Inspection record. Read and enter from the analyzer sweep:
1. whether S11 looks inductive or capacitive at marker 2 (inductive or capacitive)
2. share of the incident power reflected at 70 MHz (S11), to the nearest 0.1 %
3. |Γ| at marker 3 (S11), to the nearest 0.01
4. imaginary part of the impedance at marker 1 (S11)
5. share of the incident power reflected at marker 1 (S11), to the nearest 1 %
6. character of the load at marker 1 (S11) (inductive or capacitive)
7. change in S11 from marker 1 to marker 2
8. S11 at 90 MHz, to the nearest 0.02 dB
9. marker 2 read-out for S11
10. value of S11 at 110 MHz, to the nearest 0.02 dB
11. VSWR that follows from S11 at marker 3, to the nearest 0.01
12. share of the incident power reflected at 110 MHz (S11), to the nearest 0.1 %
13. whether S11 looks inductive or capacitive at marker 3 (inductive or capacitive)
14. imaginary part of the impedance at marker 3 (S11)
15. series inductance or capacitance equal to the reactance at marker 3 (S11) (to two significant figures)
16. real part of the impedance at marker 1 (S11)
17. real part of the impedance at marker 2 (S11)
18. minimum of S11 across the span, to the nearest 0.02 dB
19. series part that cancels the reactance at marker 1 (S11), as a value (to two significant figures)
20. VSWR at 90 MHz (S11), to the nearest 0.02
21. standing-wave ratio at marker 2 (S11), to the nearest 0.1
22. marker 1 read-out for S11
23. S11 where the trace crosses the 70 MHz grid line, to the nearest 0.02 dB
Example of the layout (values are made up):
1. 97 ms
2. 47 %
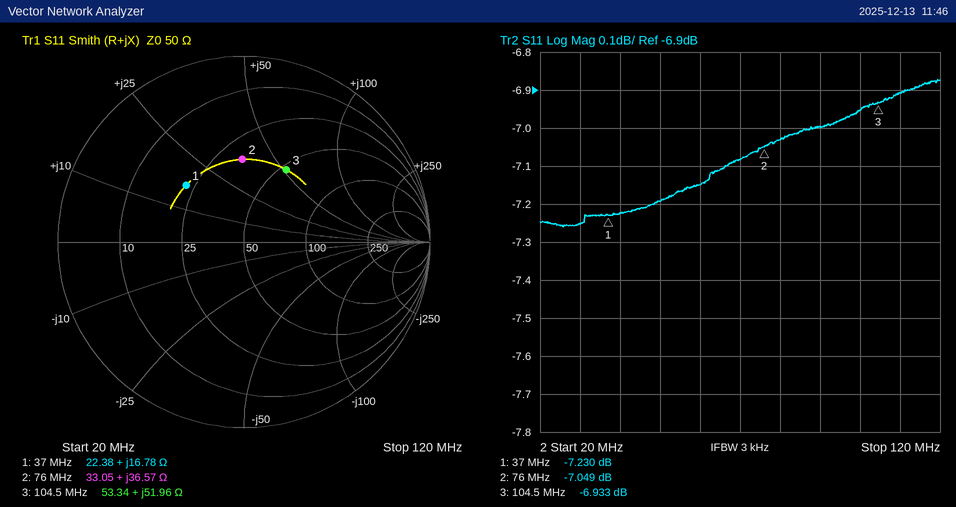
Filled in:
1. inductive
2. 19.6 %
3. 0.45
4. +16.78 Ω
5. 19 %
6. inductive
7. 0.181 dB
8. -7.00 dB
9. -7.049 dB
10. -6.90 dB
11. 2.64
12. 20.4 %
13. inductive
14. +51.96 Ω
15. 79 nH
16. 22.38 Ω
17. 33.05 Ω
18. -7.26 dB
19. 260 pF
20. 2.62
21. 2.6
22. -7.230 dB
23. -7.08 dB
